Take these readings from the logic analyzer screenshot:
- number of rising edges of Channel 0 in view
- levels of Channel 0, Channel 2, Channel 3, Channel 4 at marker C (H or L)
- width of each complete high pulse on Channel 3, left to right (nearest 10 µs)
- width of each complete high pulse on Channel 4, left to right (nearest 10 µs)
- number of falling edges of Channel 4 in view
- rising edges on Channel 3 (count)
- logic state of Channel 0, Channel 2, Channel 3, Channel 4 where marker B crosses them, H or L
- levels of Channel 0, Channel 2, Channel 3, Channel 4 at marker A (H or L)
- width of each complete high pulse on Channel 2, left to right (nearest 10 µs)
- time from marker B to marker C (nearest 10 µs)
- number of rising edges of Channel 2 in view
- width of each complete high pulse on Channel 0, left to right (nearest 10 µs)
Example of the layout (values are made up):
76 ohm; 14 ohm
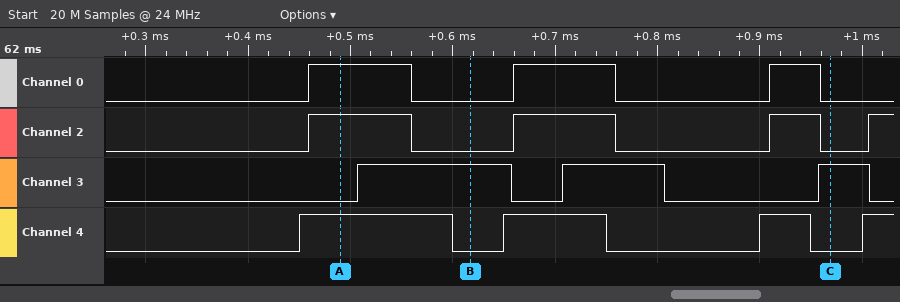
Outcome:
3; Channel 0=L, Channel 2=L, Channel 3=H, Channel 4=L; 150 µs, 100 µs, 50 µs; 150 µs, 100 µs, 50 µs; 3; 3; Channel 0=L, Channel 2=L, Channel 3=H, Channel 4=L; Channel 0=H, Channel 2=H, Channel 3=L, Channel 4=H; 100 µs, 100 µs, 50 µs; 350 µs; 4; 100 µs, 100 µs, 50 µs
